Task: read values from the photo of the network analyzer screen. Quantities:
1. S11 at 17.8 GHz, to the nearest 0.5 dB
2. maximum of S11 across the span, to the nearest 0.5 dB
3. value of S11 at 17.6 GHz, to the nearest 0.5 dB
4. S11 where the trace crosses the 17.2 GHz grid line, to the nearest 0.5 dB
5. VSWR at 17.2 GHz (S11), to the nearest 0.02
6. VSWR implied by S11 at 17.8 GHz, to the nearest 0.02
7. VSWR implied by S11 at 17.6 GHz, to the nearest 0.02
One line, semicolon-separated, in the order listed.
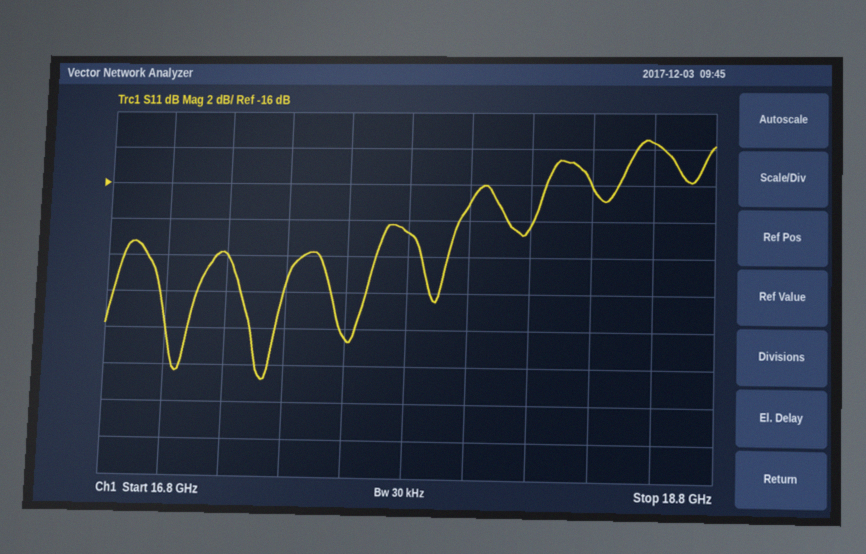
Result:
-18.5 dB; -13.5 dB; -24.5 dB; -20.0 dB; 1.22; 1.26; 1.12
